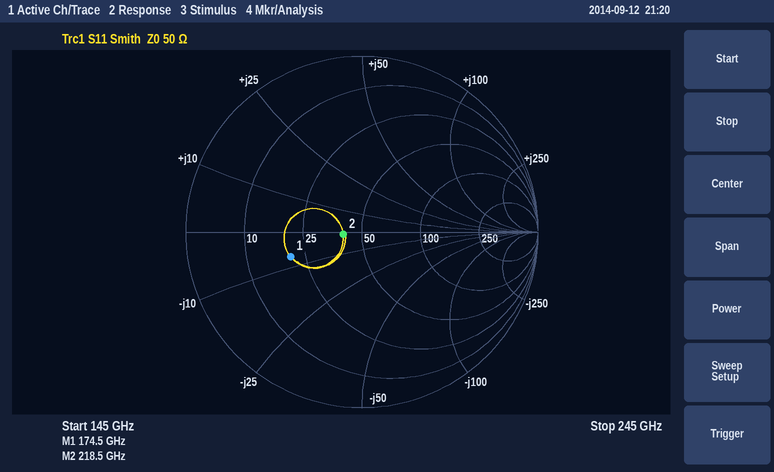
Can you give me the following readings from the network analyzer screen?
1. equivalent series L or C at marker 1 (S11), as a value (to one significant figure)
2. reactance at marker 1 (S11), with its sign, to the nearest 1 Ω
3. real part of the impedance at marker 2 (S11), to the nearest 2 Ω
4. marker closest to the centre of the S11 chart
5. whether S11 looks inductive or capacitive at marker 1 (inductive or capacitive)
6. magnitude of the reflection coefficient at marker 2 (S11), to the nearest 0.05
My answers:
100 fF
-7 Ω
40 Ω
marker 2
capacitive
0.10
